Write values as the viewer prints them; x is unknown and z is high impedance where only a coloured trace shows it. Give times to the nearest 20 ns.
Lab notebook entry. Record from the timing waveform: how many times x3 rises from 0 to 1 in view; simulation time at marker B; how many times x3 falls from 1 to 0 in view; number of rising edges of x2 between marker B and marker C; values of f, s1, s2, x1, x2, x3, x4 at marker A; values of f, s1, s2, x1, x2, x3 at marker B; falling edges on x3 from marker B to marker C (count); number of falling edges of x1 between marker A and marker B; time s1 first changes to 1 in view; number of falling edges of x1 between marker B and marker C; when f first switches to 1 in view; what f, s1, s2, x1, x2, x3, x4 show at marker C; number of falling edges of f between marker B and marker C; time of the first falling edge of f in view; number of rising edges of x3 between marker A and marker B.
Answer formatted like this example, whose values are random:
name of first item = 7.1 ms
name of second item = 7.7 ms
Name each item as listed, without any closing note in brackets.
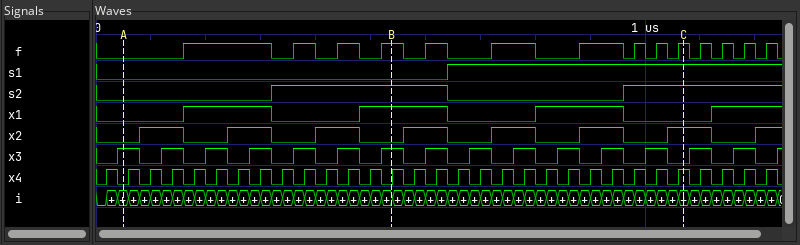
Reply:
how many times x3 rises from 0 to 1 in view = 16
simulation time at marker B = 540 ns
how many times x3 falls from 1 to 0 in view = 15
number of rising edges of x2 between marker B and marker C = 4
values of f, s1, s2, x1, x2, x3, x4 at marker A = f=0, s1=0, s2=0, x1=0, x2=0, x3=1, x4=0
values of f, s1, s2, x1, x2, x3 at marker B = f=1, s1=0, s2=1, x1=1, x2=0, x3=1
falling edges on x3 from marker B to marker C = 7
number of falling edges of x1 between marker A and marker B = 1
time s1 first changes to 1 in view = 640 ns
number of falling edges of x1 between marker B and marker C = 2
when f first switches to 1 in view = 160 ns
what f, s1, s2, x1, x2, x3, x4 show at marker C = f=1, s1=1, s2=1, x1=0, x2=1, x3=0, x4=1
number of falling edges of f between marker B and marker C = 6
time of the first falling edge of f in view = 320 ns
number of rising edges of x3 between marker A and marker B = 6
